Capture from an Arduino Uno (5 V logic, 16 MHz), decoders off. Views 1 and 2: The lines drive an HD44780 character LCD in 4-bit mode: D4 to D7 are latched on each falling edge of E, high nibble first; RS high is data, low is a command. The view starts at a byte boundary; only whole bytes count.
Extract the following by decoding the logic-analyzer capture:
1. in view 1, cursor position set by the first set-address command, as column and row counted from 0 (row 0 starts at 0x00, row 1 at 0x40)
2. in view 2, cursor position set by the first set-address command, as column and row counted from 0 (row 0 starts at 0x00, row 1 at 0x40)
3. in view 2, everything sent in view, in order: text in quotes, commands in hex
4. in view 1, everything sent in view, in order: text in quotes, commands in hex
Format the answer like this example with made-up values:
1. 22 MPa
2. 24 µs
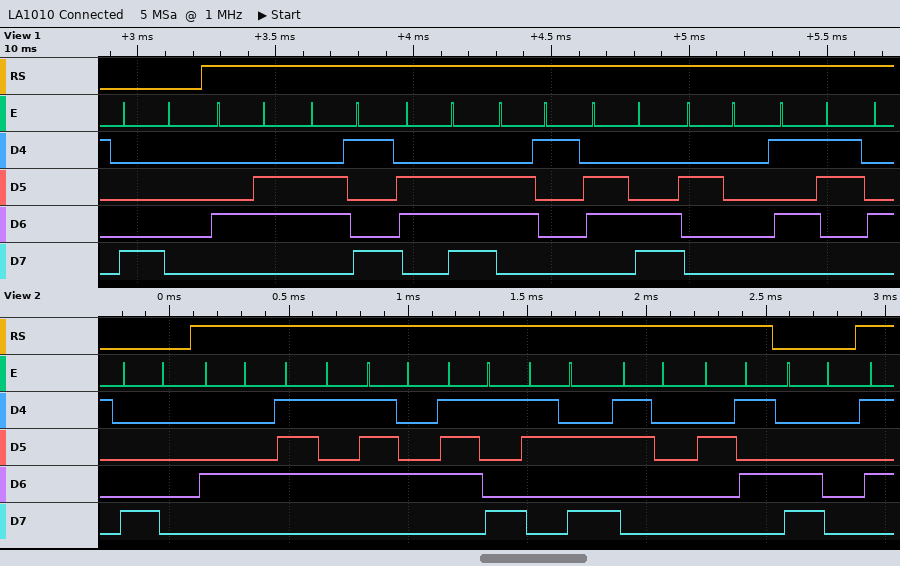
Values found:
1. column 0, row 0
2. column 0, row 0
3. 0x80 "Duty:0%" 0xC0
4. 0x80 "Final S"
